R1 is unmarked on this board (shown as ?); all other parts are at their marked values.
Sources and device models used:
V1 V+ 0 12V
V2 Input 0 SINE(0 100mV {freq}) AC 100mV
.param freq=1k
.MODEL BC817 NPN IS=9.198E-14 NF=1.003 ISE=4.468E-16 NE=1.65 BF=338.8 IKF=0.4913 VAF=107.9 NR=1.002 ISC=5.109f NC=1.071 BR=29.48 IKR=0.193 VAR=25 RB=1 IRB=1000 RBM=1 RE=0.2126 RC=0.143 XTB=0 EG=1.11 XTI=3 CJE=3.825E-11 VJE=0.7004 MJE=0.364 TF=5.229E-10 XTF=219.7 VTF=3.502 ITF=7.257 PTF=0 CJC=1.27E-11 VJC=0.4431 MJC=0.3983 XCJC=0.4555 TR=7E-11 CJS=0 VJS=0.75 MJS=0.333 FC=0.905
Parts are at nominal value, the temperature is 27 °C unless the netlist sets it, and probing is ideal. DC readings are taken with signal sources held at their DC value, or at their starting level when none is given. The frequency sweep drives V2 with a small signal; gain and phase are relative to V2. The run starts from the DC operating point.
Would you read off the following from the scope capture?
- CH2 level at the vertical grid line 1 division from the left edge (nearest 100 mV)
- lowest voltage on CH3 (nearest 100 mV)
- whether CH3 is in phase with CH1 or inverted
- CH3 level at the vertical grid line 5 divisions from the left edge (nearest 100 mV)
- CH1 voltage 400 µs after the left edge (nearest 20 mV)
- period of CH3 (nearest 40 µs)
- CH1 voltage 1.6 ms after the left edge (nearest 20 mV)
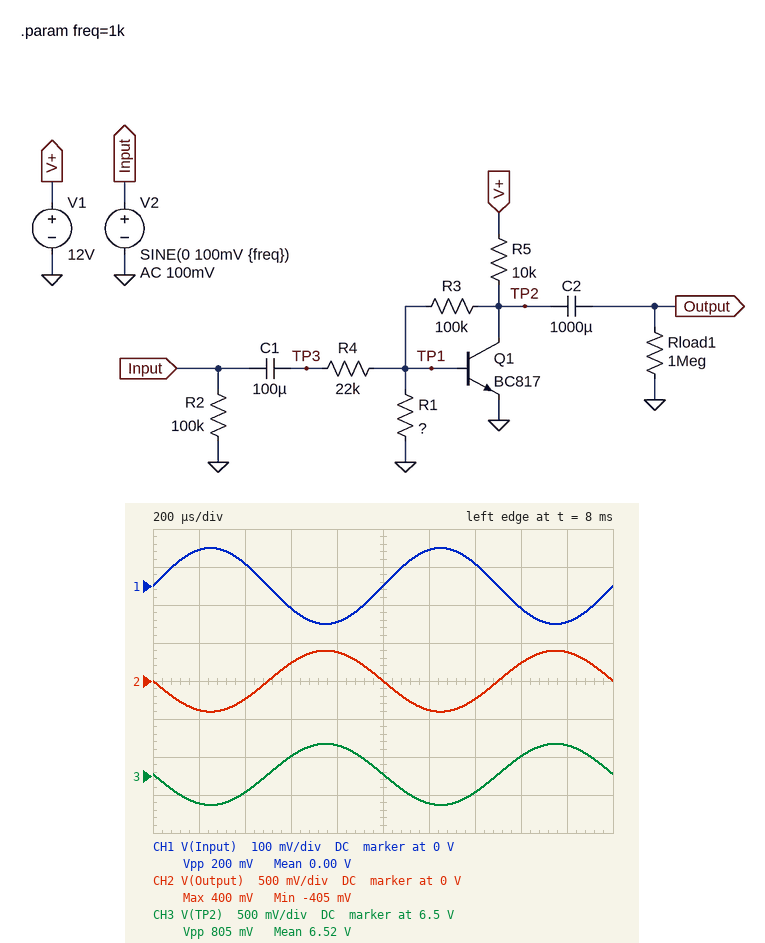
-400 mV
6.1 V
inverted
6.5 V
60 mV
1.00 ms
-60 mV
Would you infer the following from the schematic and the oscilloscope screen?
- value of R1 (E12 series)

10 kΩ
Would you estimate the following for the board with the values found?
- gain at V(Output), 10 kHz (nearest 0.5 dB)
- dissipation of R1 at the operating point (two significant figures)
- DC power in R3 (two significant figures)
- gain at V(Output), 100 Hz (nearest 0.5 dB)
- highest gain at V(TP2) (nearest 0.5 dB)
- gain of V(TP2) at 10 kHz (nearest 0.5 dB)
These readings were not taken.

12.0 dB
34 µW
350 µW
12.0 dB
12.0 dB
12.0 dB
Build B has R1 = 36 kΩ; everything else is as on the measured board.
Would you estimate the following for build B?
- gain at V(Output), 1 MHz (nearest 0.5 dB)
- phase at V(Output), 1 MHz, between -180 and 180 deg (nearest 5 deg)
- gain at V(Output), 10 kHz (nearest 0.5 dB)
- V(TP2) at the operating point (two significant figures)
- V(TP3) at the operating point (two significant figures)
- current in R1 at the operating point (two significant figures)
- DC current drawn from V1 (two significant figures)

0 dB
105 deg
12.5 dB
2.5 V
600 mV
17 µA
950 µA
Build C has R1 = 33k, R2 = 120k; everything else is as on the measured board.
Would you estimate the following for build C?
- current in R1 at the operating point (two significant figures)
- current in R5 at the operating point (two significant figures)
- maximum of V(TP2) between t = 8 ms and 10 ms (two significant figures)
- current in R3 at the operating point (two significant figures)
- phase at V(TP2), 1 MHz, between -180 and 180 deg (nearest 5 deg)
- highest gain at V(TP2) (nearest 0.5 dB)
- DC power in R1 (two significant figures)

18 µA
930 µA
3.1 V
21 µA
105 deg
12.5 dB
11 µW
